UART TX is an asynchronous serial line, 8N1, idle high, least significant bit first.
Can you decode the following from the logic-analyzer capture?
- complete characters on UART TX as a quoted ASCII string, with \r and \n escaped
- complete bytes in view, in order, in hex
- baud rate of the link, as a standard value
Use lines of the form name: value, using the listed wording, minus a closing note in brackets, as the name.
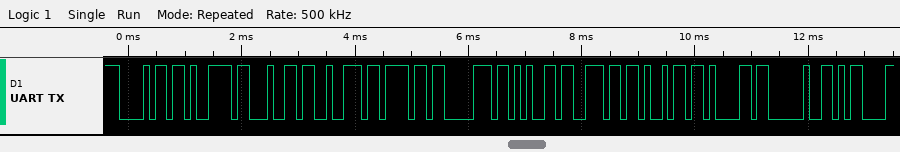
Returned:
complete characters on UART TX as a quoted ASCII string, with \r and \n escaped: "hydropenia \r"
complete bytes in view, in order, in hex: 0x68 0x79 0x64 0x72 0x6F 0x70 0x65 0x6E 0x69 0x61 0x20 0x0D
baud rate of the link, as a standard value: 9600 baud
